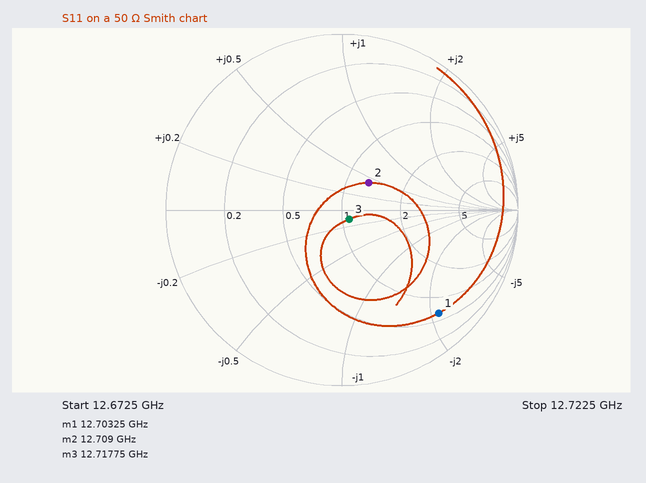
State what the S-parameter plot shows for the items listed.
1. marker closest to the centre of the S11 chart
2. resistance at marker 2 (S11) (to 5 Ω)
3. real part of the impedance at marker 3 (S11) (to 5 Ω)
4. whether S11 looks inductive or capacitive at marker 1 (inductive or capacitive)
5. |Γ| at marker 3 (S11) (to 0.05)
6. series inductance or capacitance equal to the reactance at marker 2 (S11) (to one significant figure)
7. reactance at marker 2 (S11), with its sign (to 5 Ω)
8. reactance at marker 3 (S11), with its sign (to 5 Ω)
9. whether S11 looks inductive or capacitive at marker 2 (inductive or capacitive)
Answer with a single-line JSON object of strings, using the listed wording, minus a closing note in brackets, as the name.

{"marker closest to the centre of the S11 chart": "marker 3", "resistance at marker 2 (S11)": "65 Ω", "real part of the impedance at marker 3 (S11)": "55 Ω", "whether S11 looks inductive or capacitive at marker 1": "capacitive", "|Γ| at marker 3 (S11)": "0.05", "series inductance or capacitance equal to the reactance at marker 2 (S11)": "300 pH", "reactance at marker 2 (S11), with its sign": "+20 Ω", "reactance at marker 3 (S11), with its sign": "-5 Ω", "whether S11 looks inductive or capacitive at marker 2": "inductive"}
